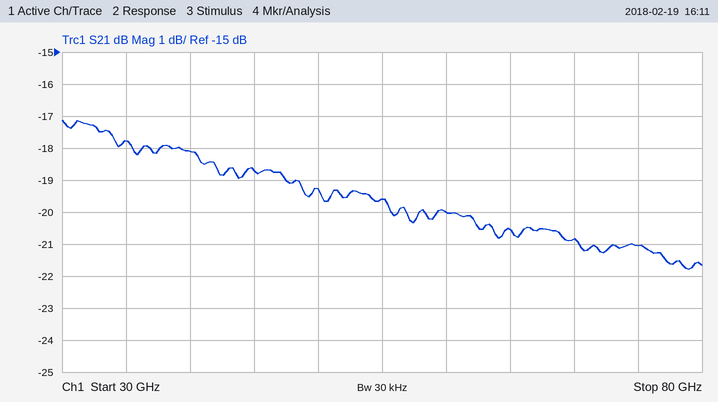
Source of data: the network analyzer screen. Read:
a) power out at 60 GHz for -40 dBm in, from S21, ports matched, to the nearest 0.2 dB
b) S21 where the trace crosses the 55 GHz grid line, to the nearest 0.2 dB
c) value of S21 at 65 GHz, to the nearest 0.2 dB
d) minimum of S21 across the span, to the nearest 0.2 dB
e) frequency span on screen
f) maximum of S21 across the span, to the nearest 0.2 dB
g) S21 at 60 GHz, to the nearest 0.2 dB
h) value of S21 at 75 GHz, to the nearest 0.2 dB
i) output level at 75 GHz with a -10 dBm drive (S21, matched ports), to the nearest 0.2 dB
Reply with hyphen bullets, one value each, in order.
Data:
- -60.0 dBm
- -19.6 dB
- -20.6 dB
- -21.8 dB
- 50 GHz
- -17.2 dB
- -20.0 dB
- -21.0 dB
- -31.0 dBm
